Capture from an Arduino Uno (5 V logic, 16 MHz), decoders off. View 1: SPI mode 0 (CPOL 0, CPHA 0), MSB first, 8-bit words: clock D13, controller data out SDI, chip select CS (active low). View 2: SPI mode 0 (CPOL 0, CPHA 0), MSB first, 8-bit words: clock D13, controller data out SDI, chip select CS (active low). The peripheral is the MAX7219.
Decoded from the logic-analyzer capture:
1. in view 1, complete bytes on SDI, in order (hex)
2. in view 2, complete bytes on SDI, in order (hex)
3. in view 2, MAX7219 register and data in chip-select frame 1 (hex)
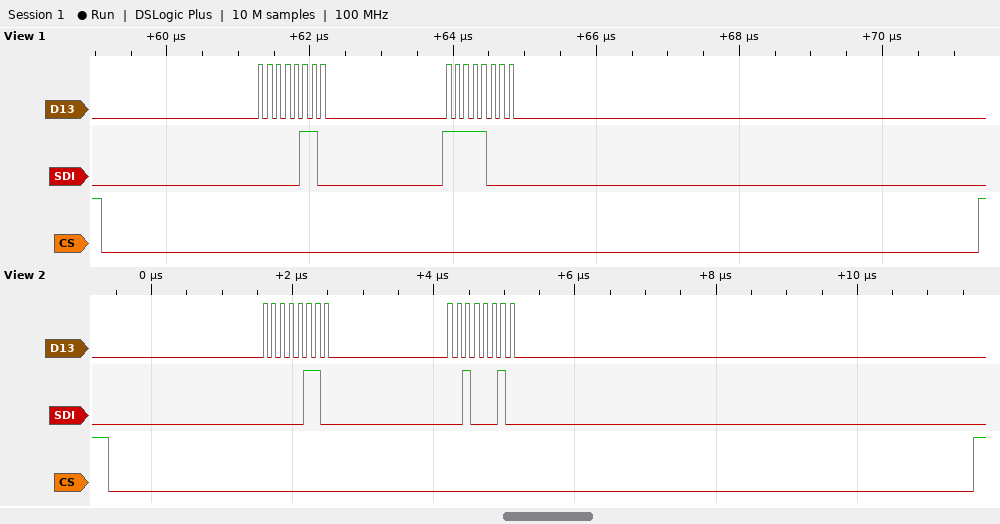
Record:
06 F8
06 22
register 0x6, data 0x22
